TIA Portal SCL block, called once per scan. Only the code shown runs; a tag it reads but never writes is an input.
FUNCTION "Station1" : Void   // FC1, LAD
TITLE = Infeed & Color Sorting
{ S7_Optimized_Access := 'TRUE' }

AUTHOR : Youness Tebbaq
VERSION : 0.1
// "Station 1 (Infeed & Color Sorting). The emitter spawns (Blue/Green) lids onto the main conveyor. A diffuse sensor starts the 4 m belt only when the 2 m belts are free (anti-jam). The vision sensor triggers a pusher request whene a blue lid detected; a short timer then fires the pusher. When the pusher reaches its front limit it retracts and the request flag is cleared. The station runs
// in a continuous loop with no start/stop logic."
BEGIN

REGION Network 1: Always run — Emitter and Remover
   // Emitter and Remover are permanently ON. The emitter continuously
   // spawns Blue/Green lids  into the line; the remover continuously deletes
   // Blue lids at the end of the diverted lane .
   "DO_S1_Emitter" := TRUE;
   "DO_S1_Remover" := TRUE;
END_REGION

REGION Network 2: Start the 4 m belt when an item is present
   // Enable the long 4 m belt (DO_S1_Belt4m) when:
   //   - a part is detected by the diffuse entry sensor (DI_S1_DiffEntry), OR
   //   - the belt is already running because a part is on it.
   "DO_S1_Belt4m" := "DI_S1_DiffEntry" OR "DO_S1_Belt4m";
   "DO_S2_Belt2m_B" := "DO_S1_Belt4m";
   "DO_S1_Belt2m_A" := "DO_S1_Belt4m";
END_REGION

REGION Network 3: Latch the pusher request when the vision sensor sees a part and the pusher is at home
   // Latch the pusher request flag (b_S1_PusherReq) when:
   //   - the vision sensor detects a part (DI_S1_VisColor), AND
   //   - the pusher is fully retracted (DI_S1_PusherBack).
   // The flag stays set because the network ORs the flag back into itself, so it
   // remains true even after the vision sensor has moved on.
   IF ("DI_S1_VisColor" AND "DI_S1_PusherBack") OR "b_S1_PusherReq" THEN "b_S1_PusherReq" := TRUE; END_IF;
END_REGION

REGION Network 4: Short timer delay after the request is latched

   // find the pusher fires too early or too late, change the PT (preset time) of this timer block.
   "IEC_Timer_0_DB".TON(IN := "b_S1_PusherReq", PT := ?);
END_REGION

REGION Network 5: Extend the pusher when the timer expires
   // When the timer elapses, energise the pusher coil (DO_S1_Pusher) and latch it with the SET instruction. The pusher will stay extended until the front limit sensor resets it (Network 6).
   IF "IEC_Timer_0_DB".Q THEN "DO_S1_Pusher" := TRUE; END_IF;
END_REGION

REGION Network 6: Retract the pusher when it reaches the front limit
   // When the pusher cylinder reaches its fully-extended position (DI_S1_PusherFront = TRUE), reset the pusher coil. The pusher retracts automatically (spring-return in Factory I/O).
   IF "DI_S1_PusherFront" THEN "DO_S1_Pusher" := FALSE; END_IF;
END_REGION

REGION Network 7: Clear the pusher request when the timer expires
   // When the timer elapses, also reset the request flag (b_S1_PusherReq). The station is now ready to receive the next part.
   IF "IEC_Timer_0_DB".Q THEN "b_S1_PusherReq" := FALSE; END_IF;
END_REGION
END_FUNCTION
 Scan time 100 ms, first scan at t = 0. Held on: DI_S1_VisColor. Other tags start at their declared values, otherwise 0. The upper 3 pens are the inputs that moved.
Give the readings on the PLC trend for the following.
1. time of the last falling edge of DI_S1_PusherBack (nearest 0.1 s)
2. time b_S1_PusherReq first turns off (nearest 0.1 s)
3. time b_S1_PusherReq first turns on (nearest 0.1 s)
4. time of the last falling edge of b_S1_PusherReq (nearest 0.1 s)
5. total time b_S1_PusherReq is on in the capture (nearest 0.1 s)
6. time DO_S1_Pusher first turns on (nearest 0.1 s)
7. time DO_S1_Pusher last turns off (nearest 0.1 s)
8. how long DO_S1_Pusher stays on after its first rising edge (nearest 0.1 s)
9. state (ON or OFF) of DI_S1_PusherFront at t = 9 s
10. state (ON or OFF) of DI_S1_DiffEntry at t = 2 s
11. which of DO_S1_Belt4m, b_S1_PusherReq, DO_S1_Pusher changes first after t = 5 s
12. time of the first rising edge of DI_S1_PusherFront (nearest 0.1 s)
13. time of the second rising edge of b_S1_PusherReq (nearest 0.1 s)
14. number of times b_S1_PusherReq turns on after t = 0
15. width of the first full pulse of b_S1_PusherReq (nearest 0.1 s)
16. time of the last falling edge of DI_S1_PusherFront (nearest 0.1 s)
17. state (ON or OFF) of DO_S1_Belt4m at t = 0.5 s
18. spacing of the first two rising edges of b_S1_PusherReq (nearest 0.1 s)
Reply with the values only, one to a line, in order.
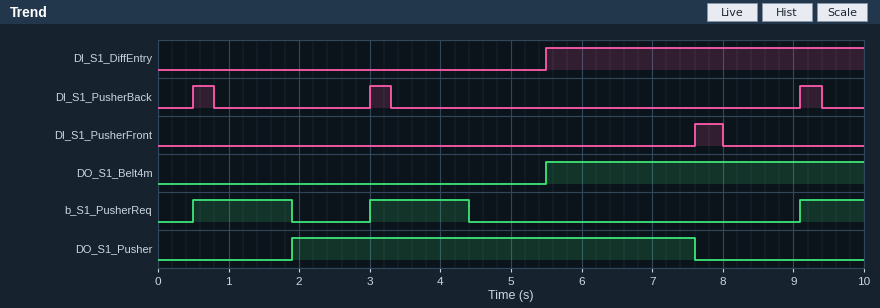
9.4 s
1.9 s
0.5 s
4.4 s
3.7 s
1.9 s
7.6 s
5.7 s
OFF
OFF
DO_S1_Belt4m
7.6 s
3.0 s
3
1.4 s
8.0 s
OFF
2.5 s
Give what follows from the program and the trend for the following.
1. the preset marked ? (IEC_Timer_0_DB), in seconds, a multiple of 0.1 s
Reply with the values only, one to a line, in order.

1.4 s
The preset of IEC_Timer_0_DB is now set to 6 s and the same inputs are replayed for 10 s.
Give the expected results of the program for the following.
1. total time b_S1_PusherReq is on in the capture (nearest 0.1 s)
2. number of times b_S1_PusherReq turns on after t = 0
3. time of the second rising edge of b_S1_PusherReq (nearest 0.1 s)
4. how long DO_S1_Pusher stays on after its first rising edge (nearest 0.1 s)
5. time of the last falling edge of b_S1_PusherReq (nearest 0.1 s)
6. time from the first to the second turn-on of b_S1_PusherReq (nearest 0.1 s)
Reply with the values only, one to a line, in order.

6.9 s
2
9.1 s
1.1 s
6.5 s
8.6 s
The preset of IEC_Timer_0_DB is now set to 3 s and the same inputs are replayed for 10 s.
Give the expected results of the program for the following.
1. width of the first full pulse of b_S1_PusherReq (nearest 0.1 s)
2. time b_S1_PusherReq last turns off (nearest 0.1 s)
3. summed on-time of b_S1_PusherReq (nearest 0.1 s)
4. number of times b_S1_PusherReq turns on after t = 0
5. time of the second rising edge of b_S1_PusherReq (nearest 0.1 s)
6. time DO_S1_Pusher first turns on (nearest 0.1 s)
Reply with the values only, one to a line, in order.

3.0 s
3.5 s
3.9 s
2
9.1 s
3.5 s
